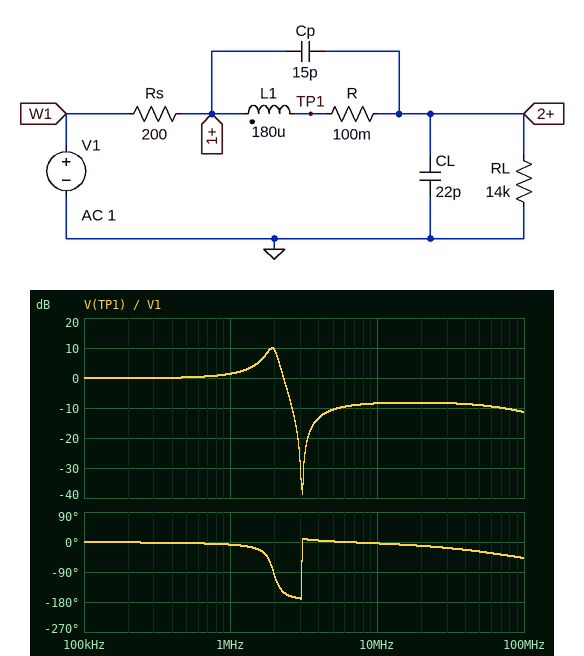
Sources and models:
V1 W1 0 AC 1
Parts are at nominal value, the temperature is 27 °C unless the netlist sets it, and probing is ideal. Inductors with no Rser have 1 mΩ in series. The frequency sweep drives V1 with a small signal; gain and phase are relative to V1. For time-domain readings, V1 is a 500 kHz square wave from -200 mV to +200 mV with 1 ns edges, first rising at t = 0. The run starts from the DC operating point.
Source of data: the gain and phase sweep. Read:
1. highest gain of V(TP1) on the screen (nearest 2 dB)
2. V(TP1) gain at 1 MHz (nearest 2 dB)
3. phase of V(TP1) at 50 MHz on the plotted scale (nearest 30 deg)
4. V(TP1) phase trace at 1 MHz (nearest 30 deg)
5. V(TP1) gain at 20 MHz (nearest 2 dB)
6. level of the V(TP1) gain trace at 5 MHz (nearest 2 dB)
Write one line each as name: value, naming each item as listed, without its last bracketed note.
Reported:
highest gain of V(TP1) on the screen: 10 dB
V(TP1) gain at 1 MHz: 2 dB
phase of V(TP1) at 50 MHz on the plotted scale: -30 deg
V(TP1) phase trace at 1 MHz: 0 deg
V(TP1) gain at 20 MHz: -8 dB
level of the V(TP1) gain trace at 5 MHz: -10 dB
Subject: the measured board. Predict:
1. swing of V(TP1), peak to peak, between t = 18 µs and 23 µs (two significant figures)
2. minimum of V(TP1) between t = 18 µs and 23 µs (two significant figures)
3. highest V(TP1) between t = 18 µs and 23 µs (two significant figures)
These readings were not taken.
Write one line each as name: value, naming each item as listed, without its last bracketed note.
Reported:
swing of V(TP1), peak to peak, between t = 18 µs and 23 µs: 660 mV
minimum of V(TP1) between t = 18 µs and 23 µs: -330 mV
highest V(TP1) between t = 18 µs and 23 µs: 330 mV
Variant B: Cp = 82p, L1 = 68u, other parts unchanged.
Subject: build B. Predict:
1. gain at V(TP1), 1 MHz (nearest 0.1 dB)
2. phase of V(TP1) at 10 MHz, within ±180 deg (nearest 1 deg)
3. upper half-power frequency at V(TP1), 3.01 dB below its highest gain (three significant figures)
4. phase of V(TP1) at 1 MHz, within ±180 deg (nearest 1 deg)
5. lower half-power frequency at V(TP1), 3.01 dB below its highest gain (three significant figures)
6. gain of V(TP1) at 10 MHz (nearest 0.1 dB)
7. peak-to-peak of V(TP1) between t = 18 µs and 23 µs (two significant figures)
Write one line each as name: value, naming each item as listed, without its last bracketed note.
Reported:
gain at V(TP1), 1 MHz: 0.5 dB
phase of V(TP1) at 10 MHz, within ±180 deg: -11 deg
upper half-power frequency at V(TP1), 3.01 dB below its highest gain: 1.93 MHz
phase of V(TP1) at 1 MHz, within ±180 deg: -4 deg
lower half-power frequency at V(TP1), 3.01 dB below its highest gain: 1.78 MHz
gain of V(TP1) at 10 MHz: -2.4 dB
peak-to-peak of V(TP1) between t = 18 µs and 23 µs: 490 mV
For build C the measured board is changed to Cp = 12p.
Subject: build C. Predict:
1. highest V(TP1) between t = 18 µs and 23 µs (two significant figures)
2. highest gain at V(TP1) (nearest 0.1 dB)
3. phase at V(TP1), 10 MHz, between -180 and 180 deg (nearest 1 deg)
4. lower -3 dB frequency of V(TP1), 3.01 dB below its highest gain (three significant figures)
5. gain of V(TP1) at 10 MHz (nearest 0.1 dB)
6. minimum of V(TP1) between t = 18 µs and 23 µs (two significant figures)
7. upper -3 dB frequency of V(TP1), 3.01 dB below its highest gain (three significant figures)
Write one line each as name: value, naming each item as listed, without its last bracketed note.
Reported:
highest V(TP1) between t = 18 µs and 23 µs: 340 mV
highest gain at V(TP1): 10.2 dB
phase at V(TP1), 10 MHz, between -180 and 180 deg: -3 deg
lower -3 dB frequency of V(TP1), 3.01 dB below its highest gain: 1.75 MHz
gain of V(TP1) at 10 MHz: -9.8 dB
minimum of V(TP1) between t = 18 µs and 23 µs: -340 mV
upper -3 dB frequency of V(TP1), 3.01 dB below its highest gain: 2.19 MHz
